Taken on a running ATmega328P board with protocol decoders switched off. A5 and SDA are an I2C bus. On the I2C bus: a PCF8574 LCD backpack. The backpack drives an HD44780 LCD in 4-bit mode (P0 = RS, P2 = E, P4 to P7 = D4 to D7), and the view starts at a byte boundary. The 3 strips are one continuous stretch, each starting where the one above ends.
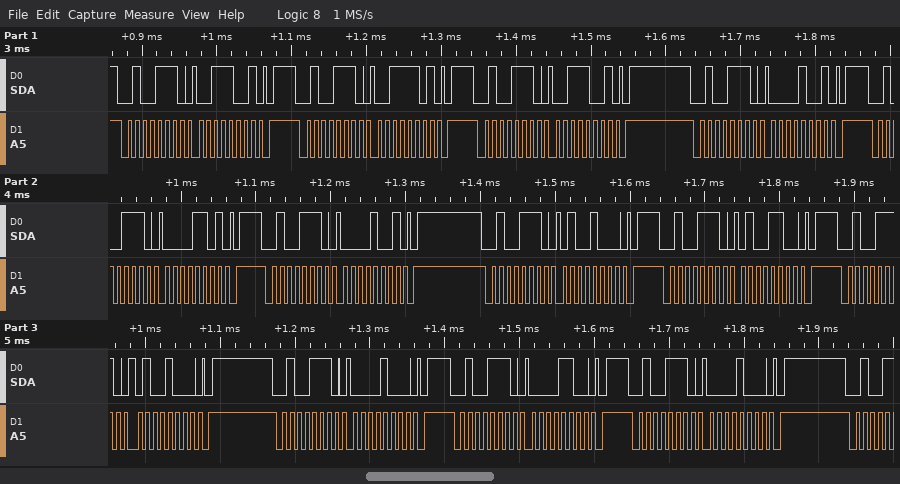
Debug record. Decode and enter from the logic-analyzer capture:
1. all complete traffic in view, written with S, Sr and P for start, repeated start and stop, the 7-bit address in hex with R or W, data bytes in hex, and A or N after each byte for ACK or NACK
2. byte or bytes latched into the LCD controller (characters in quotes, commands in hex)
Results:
S 27W A 39 A P S 27W A 3D A P S 27W A 39 A P S 27W A 09 A P S 27W A 0D A P S 27W A 09 A P S 27W A 48 A P S 27W A 4C A P S 27W A 48 A P S 27W A 08 A P S 27W A 0C A P S 27W A 08 A P
'0' 0x40
